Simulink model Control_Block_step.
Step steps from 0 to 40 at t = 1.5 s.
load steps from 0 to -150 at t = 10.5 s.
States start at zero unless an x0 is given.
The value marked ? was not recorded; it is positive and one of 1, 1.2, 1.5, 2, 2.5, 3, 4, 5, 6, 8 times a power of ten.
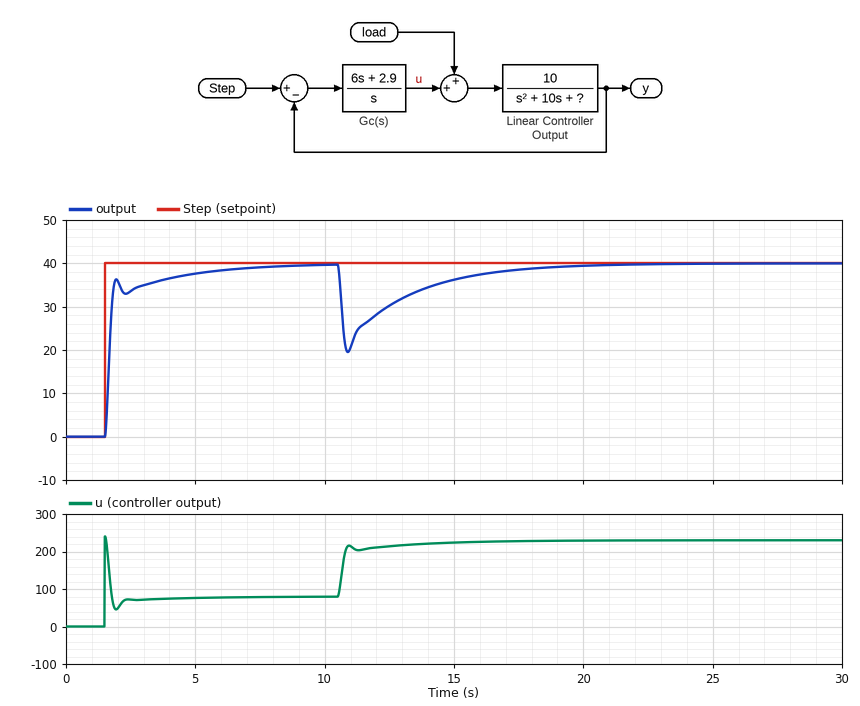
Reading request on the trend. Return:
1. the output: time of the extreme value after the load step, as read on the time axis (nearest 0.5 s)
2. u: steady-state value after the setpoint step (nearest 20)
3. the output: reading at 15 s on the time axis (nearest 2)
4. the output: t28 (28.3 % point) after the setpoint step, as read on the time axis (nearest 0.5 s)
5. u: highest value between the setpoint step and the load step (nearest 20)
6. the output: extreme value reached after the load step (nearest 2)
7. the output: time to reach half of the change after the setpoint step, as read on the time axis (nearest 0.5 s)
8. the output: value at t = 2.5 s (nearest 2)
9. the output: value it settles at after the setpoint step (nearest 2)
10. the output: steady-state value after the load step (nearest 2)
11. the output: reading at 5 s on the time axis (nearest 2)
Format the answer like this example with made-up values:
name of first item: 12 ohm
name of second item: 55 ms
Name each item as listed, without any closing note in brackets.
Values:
the output: time of the extreme value after the load step, as read on the time axis: 11.0 s
u: steady-state value after the setpoint step: 80
the output: reading at 15 s on the time axis: 36
the output: t28 (28.3 % point) after the setpoint step, as read on the time axis: 1.5 s
u: highest value between the setpoint step and the load step: 240
the output: extreme value reached after the load step: 20
the output: time to reach half of the change after the setpoint step, as read on the time axis: 1.5 s
the output: value at t = 2.5 s: 34
the output: value it settles at after the setpoint step: 40
the output: steady-state value after the load step: 40
the output: reading at 5 s on the time axis: 38
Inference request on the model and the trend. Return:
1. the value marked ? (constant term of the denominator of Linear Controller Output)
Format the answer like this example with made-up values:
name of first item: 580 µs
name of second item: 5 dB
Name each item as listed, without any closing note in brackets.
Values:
the value marked ?: 20
